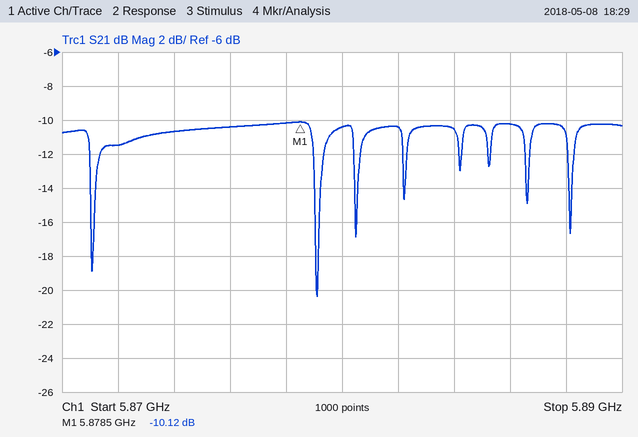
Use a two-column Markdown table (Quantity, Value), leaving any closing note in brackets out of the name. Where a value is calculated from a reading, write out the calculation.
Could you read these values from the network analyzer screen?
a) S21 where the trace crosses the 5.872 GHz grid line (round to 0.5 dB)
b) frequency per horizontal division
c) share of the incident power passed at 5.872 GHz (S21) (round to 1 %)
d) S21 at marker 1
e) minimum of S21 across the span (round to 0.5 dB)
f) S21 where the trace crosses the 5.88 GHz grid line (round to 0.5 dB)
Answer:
| Quantity | Value |
|---|---|
| S21 where the trace crosses the 5.872 GHz grid line | -11.5 dB |
| frequency per horizontal division | 2 MHz |
| share of the incident power passed at 5.872 GHz (S21) | 10^(-11.5/10) ≈ 7 % |
| S21 at marker 1 | -10.12 dB |
| minimum of S21 across the span | -20.5 dB |
| S21 where the trace crosses the 5.88 GHz grid line | -10.5 dB |
